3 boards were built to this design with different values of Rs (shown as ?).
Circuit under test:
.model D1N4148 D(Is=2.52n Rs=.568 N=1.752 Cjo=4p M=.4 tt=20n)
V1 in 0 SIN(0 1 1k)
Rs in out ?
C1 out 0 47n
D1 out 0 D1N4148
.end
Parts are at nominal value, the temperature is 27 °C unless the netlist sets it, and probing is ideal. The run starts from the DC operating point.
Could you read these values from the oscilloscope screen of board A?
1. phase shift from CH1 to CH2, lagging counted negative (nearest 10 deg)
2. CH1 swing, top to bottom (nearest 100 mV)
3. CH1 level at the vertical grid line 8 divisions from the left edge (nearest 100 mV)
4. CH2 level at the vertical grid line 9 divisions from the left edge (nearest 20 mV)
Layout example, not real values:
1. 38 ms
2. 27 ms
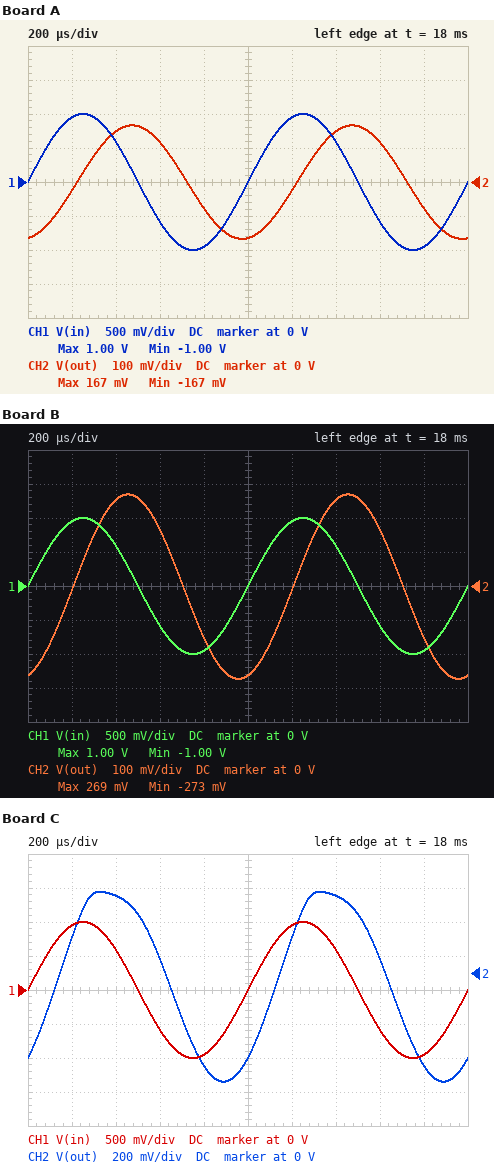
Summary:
1. -80 deg
2. 2.0 V
3. -600 mV
4. -80 mV
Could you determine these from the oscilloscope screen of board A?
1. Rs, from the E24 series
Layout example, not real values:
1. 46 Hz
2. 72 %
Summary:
1. 20 kΩ
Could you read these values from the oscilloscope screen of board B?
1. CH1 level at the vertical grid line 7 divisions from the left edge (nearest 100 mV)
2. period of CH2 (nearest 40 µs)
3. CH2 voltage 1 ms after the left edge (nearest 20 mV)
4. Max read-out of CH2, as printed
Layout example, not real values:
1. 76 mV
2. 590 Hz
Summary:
1. 600 mV
2. 1.00 ms
3. -260 mV
4. 269 mV
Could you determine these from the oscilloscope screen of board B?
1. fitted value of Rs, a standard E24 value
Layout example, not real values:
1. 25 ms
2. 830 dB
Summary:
1. 12 kΩ
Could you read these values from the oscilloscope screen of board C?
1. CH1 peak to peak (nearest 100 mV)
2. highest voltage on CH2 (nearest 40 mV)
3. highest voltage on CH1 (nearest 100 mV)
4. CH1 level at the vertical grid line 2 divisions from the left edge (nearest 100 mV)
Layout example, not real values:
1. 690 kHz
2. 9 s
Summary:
1. 2.0 V
2. 480 mV
3. 1.0 V
4. 600 mV
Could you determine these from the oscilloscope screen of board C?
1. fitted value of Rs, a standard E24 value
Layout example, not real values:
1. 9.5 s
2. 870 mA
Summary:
1. 4.3 kΩ
